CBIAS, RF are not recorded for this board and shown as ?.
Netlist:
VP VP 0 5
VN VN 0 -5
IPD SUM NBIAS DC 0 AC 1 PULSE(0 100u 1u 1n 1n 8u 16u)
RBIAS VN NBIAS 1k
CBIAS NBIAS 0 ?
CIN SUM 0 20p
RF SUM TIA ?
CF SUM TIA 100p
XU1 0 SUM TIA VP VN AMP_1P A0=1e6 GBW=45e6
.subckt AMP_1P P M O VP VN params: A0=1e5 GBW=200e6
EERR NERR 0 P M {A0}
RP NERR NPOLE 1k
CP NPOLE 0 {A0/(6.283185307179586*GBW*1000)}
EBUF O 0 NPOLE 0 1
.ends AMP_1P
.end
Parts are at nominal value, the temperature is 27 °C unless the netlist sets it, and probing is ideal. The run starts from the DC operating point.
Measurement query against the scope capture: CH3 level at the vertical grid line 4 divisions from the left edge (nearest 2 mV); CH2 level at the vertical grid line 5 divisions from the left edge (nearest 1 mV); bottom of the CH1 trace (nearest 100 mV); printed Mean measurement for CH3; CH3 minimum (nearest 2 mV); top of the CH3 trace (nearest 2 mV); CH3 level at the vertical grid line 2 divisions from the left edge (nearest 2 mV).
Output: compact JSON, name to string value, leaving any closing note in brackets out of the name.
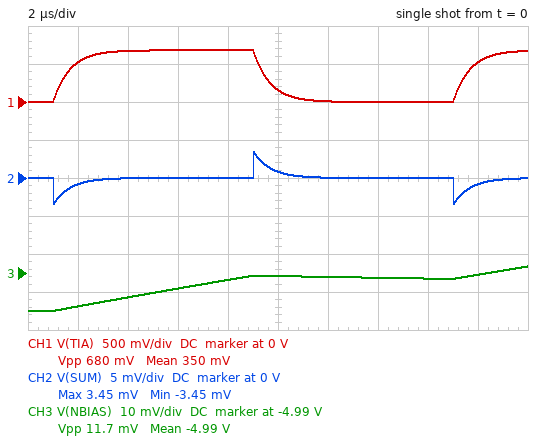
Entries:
{"CH3 level at the vertical grid line 4 divisions from the left edge": "-4.992 V", "CH2 level at the vertical grid line 5 divisions from the left edge": "1 mV", "bottom of the CH1 trace": "0 V", "printed Mean measurement for CH3": "-4.99 V", "CH3 minimum": "-5.000 V", "top of the CH3 trace": "-4.988 V", "CH3 level at the vertical grid line 2 divisions from the left edge": "-4.996 V"}
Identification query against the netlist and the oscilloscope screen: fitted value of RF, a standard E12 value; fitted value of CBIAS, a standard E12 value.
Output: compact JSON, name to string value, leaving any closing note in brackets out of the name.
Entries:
{"fitted value of RF, a standard E12 value": "6.8 kΩ", "fitted value of CBIAS, a standard E12 value": "82 nF"}
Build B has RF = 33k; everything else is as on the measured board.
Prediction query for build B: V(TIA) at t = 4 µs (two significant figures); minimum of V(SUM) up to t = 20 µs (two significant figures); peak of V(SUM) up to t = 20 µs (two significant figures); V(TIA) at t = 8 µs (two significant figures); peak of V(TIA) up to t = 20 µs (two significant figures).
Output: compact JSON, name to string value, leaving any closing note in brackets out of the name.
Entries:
{"V(TIA) at t = 4 µs": "2.0 V", "minimum of V(SUM) up to t = 20 µs": "-3.5 mV", "peak of V(SUM) up to t = 20 µs": "3.2 mV", "V(TIA) at t = 8 µs": "2.9 V", "peak of V(TIA) up to t = 20 µs": "3.0 V"}
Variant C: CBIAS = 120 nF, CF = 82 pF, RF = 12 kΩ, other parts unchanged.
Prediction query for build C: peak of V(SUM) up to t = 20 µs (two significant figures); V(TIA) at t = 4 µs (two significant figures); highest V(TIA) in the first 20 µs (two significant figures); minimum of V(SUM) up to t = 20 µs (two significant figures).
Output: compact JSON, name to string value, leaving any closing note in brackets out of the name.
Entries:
{"peak of V(SUM) up to t = 20 µs": "4.2 mV", "V(TIA) at t = 4 µs": "1.1 V", "highest V(TIA) in the first 20 µs": "1.2 V", "minimum of V(SUM) up to t = 20 µs": "-4.2 mV"}
